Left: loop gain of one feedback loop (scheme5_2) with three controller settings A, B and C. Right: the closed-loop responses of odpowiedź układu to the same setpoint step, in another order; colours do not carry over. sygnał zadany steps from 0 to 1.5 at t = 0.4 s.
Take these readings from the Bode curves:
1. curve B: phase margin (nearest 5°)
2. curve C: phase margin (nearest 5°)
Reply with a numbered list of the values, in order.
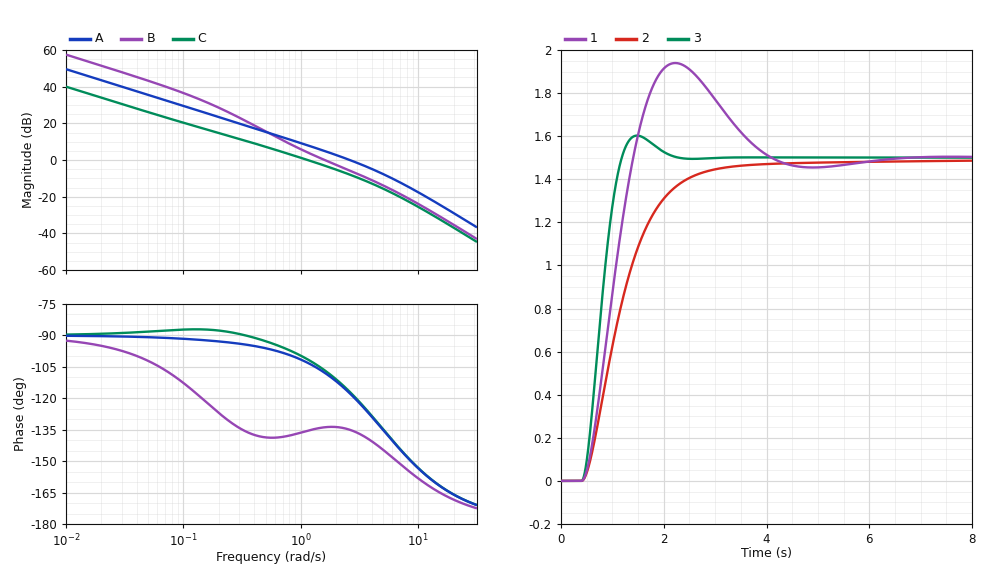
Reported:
1. 45°
2. 80°
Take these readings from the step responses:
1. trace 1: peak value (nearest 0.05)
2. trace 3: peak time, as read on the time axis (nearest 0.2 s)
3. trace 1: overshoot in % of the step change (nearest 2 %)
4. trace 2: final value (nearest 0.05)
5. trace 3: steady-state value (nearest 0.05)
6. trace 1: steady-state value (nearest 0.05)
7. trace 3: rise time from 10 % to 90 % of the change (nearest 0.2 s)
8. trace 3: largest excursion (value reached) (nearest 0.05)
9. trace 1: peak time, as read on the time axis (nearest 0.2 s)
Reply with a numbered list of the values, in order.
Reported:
1. 1.95
2. 1.4 s
3. 30 %
4. 1.50
5. 1.50
6. 1.50
7. 0.6 s
8. 1.60
9. 2.2 s
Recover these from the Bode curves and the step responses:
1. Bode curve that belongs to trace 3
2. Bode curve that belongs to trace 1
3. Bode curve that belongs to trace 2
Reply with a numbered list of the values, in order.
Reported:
1. A
2. B
3. C
